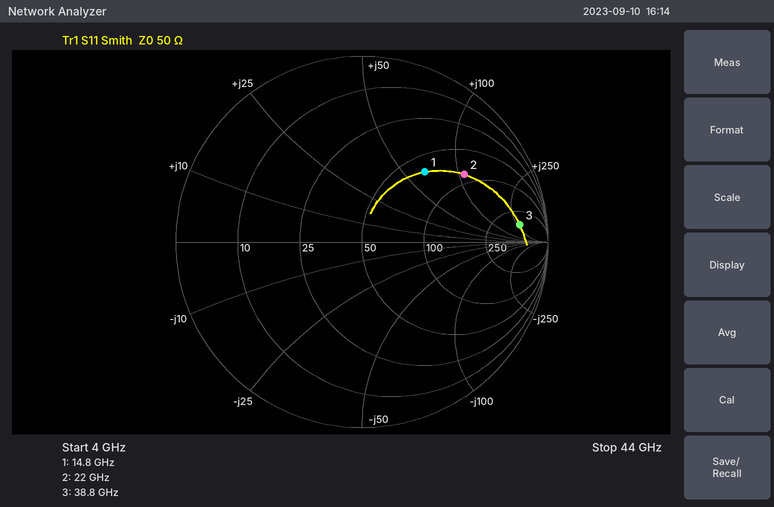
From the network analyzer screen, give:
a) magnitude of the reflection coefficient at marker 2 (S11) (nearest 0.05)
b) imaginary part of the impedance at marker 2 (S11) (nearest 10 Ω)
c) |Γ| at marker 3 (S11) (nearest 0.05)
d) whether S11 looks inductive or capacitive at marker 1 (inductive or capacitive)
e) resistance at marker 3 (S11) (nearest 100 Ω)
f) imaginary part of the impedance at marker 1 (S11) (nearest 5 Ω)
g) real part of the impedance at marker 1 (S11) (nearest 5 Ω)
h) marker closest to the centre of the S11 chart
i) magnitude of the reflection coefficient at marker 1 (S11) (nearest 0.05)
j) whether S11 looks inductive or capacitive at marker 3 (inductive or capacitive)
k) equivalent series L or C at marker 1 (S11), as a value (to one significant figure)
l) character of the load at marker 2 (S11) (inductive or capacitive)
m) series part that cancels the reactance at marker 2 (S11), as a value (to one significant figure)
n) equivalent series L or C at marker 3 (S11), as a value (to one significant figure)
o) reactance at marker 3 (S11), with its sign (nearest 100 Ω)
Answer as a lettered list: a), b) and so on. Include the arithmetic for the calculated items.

a) 0.65
b) +110 Ω
c) 0.85
d) inductive
e) 400 Ω
f) +65 Ω
g) 65 Ω
h) marker 1
i) 0.50
j) inductive
k) L = 65 Ω/(2π × 14.8 GHz) ≈ 699 pH, so 700 pH to one significant figure
l) inductive
m) C = 1/(2π × 22 GHz × 110 Ω) ≈ 65.8 fF, so 70 fF to one significant figure
n) L = 300 Ω/(2π × 38.8 GHz) ≈ 1 nH
o) +300 Ω
